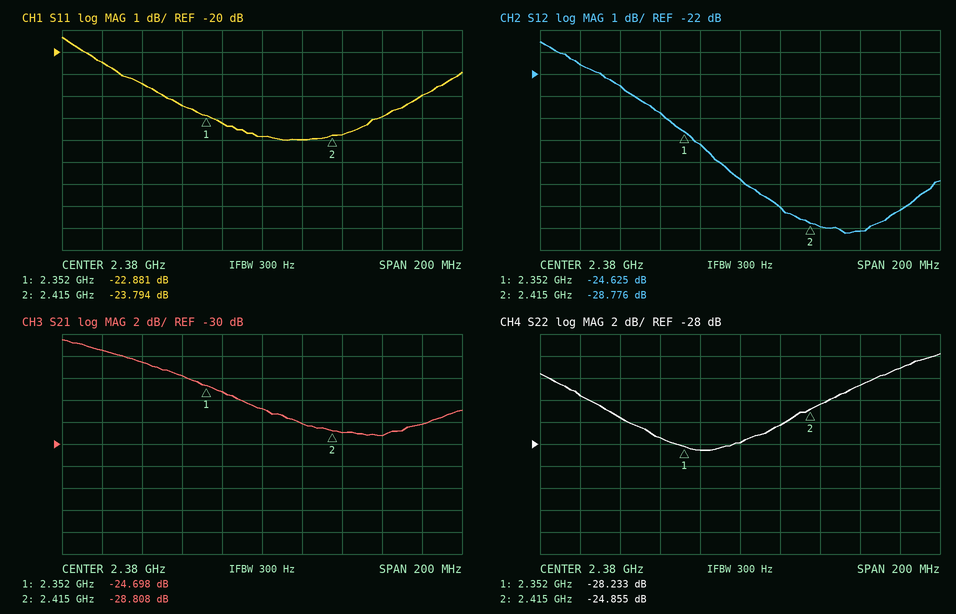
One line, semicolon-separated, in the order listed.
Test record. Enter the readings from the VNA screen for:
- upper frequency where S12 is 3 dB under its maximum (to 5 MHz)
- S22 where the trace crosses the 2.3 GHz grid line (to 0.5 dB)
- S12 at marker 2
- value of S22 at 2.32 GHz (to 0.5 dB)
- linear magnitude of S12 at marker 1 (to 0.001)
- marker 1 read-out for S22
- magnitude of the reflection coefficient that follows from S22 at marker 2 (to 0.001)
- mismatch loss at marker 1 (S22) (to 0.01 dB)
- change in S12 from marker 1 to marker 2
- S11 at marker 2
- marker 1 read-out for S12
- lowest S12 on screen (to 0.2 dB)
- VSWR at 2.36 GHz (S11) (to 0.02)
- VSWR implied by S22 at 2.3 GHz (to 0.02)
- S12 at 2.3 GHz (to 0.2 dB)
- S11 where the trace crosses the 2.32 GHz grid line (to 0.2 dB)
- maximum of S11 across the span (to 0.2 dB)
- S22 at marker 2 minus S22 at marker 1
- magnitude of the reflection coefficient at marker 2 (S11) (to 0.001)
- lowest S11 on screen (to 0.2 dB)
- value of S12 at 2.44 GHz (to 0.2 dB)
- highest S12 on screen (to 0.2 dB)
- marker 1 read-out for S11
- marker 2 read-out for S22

2.335 GHz; -23.5 dB; -28.776 dB; -25.5 dB; 0.059; -28.233 dB; 0.057; 0.01 dB; -4.151 dB; -23.794 dB; -24.625 dB; -29.2 dB; 1.14; 1.14; -21.6 dB; -21.4 dB; -19.4 dB; 3.378 dB; 0.065; -24.0 dB; -29.2 dB; -20.6 dB; -22.881 dB; -24.855 dB
